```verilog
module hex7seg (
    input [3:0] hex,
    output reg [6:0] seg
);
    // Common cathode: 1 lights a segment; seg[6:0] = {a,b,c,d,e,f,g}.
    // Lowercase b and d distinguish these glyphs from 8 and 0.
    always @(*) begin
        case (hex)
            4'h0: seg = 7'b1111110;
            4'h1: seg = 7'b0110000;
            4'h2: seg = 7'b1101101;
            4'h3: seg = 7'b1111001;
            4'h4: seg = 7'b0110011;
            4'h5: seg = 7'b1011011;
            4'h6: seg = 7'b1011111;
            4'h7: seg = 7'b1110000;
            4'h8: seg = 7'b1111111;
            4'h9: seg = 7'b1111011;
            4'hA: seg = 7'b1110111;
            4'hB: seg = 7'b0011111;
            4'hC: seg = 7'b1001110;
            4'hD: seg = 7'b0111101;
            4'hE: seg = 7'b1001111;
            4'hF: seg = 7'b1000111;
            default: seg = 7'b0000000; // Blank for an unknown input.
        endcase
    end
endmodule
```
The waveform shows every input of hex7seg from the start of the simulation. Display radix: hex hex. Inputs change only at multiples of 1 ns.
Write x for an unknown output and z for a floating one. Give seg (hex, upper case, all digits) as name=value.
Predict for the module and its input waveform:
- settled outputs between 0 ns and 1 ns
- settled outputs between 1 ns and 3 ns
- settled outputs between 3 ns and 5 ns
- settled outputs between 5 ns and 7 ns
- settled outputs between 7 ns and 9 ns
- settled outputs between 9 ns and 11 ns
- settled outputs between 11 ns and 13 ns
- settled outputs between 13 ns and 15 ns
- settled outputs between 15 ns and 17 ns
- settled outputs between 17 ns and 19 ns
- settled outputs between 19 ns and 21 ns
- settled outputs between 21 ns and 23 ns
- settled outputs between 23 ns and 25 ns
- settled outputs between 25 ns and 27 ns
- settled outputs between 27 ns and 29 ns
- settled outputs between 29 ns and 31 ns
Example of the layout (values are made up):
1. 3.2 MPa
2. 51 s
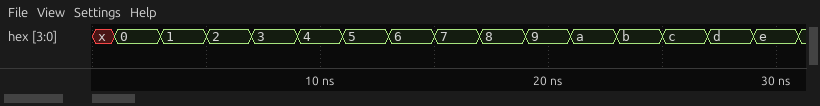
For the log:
1. seg=x
2. seg=7E
3. seg=30
4. seg=6D
5. seg=79
6. seg=33
7. seg=5B
8. seg=5F
9. seg=70
10. seg=7F
11. seg=7B
12. seg=77
13. seg=1F
14. seg=4E
15. seg=3D
16. seg=4F
